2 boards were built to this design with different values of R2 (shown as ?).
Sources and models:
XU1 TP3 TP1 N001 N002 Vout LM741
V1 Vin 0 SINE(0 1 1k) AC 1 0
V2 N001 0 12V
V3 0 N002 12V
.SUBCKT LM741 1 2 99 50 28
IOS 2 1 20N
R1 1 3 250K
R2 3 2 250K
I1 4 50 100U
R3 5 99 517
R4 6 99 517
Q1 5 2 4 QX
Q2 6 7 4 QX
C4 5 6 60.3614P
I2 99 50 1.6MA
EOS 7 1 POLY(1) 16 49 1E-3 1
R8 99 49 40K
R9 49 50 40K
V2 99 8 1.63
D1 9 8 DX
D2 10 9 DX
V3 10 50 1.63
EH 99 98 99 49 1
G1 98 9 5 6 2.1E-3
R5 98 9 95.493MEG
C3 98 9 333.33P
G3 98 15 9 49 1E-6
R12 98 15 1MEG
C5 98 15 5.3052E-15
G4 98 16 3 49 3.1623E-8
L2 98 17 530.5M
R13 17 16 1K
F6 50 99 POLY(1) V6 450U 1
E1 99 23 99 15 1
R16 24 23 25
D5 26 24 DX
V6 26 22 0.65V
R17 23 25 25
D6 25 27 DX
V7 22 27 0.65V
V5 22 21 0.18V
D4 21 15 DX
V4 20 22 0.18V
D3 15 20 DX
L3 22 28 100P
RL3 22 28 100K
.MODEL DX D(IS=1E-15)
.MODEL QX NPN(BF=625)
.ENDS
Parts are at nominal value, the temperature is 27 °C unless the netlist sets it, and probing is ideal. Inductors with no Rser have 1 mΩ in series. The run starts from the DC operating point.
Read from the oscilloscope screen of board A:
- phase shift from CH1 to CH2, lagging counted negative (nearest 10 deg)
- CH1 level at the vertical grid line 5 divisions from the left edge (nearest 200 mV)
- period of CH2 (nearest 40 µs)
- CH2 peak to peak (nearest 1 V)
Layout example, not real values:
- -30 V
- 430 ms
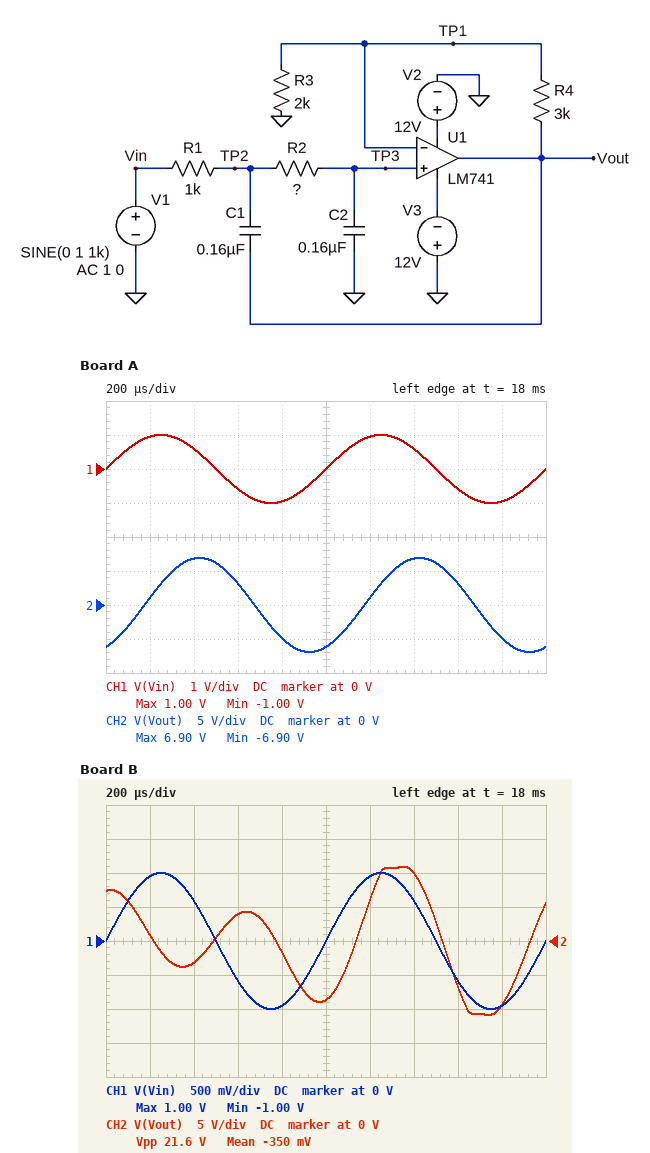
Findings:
- -60 deg
- 0 V
- 1.00 ms
- 14 V
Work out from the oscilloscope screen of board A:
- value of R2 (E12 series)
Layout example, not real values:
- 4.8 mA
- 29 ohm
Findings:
- 820 Ω
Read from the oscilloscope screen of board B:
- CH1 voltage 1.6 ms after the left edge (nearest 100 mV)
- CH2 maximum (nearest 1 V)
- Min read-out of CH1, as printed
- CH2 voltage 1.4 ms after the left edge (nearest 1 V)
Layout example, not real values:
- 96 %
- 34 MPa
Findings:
- -600 mV
- 11 V
- -1.00 V
- 10 V
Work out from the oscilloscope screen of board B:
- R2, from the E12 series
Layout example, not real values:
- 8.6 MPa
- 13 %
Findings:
- 470 Ω
